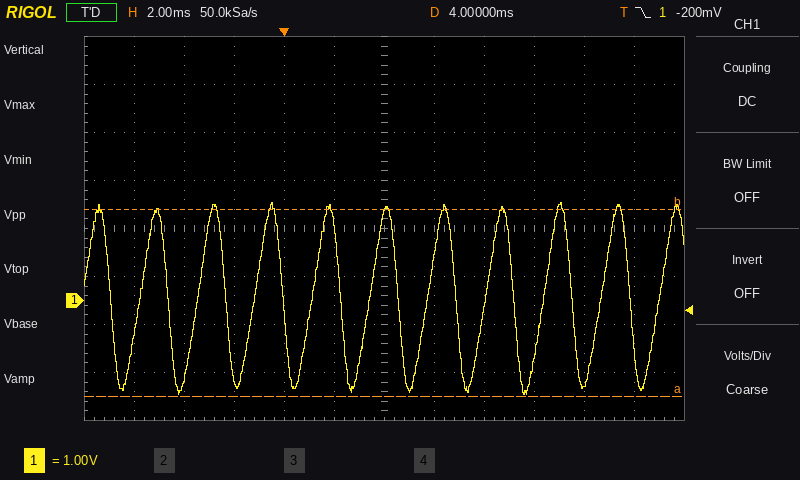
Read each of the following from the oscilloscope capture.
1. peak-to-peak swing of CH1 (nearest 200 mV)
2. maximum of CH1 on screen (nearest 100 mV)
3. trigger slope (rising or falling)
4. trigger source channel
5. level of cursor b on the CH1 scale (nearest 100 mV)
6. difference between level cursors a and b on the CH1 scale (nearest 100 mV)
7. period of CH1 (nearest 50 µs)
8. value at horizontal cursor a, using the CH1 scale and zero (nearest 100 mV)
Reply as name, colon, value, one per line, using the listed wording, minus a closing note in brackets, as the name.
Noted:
peak-to-peak swing of CH1: 4.0 V
maximum of CH1 on screen: 2.0 V
trigger slope: falling
trigger source channel: CH1
level of cursor b on the CH1 scale: 1.9 V
difference between level cursors a and b on the CH1 scale: 3.9 V
period of CH1: 2.30 ms
value at horizontal cursor a, using the CH1 scale and zero: -2.0 V
